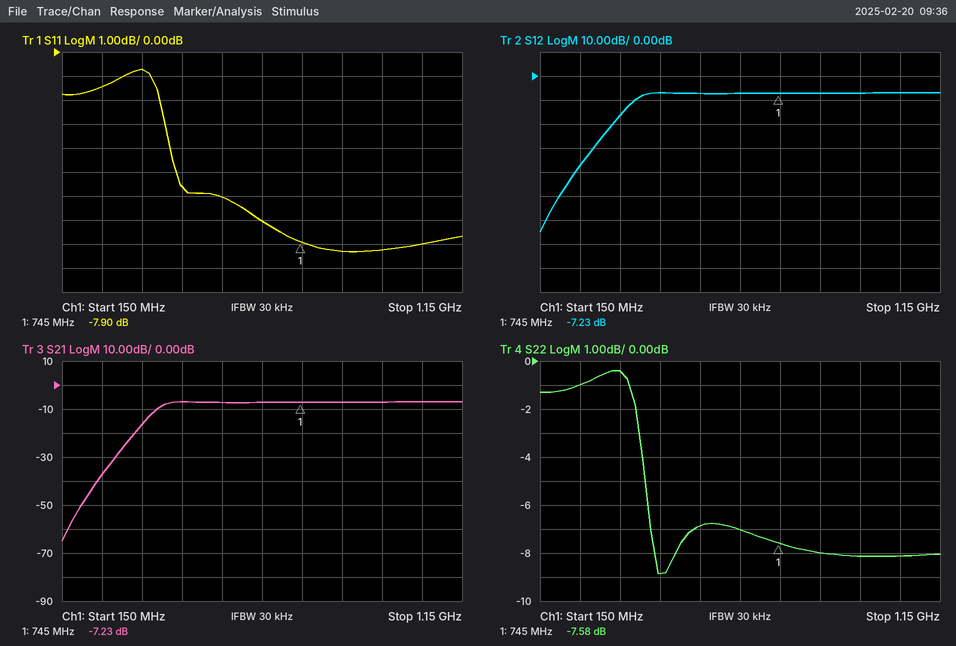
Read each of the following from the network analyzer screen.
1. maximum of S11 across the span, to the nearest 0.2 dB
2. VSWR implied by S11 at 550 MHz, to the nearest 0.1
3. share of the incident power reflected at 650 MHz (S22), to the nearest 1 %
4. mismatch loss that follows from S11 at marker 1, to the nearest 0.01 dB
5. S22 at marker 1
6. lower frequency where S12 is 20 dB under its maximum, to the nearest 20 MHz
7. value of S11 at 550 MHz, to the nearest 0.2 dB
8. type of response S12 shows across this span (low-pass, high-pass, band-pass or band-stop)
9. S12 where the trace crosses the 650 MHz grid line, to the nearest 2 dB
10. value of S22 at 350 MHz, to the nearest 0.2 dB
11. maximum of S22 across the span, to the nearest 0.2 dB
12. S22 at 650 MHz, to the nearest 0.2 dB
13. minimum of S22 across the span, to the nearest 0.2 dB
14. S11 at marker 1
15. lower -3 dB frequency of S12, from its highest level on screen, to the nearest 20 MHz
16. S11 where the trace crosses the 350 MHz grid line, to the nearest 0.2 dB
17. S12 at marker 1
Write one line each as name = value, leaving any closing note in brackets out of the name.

maximum of S11 across the span, to the nearest 0.2 dB = -0.8 dB
VSWR implied by S11 at 550 MHz, to the nearest 0.1 = 3.0
share of the incident power reflected at 650 MHz (S22), to the nearest 1 % = 20 %
mismatch loss that follows from S11 at marker 1, to the nearest 0.01 dB = 0.77 dB
S22 at marker 1 = -7.58 dB
lower frequency where S12 is 20 dB under its maximum, to the nearest 20 MHz = 300 MHz
value of S11 at 550 MHz, to the nearest 0.2 dB = -6.0 dB
type of response S12 shows across this span = high-pass
S12 where the trace crosses the 650 MHz grid line, to the nearest 2 dB = -8 dB
value of S22 at 350 MHz, to the nearest 0.2 dB = -0.4 dB
maximum of S22 across the span, to the nearest 0.2 dB = -0.4 dB
S22 at 650 MHz, to the nearest 0.2 dB = -7.0 dB
minimum of S22 across the span, to the nearest 0.2 dB = -8.8 dB
S11 at marker 1 = -7.90 dB
lower -3 dB frequency of S12, from its highest level on screen, to the nearest 20 MHz = 380 MHz
S11 where the trace crosses the 350 MHz grid line, to the nearest 0.2 dB = -0.8 dB
S12 at marker 1 = -7.23 dB
